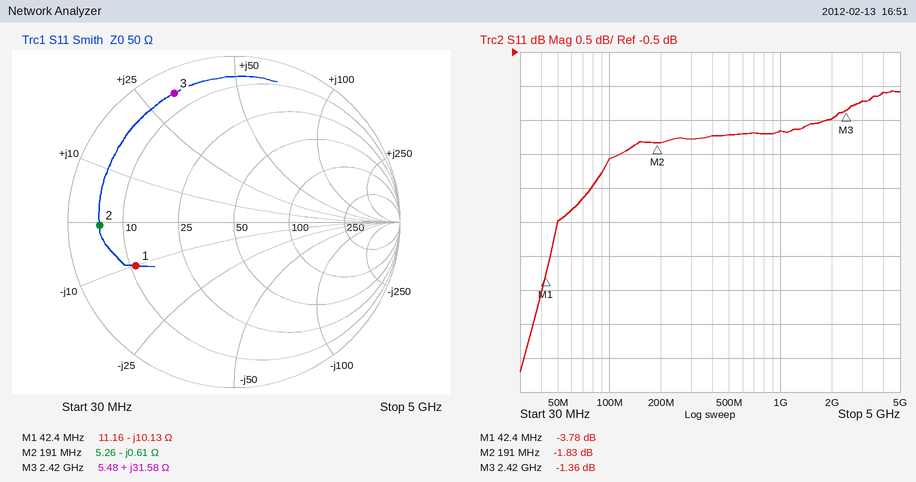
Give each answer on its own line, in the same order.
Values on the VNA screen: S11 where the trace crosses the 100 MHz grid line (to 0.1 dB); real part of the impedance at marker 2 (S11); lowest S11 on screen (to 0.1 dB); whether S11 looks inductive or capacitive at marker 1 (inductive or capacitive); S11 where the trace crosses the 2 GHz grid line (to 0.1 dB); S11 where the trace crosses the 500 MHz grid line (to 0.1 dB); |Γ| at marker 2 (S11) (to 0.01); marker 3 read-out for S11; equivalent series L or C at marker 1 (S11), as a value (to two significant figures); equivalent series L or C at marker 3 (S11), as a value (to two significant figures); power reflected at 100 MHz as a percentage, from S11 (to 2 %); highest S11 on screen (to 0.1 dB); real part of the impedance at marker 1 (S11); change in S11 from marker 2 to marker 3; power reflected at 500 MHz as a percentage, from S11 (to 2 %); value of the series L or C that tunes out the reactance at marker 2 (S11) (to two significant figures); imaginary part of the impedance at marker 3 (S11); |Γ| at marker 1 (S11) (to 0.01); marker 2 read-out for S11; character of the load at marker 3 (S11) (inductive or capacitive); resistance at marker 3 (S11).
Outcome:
-2.1 dB
5.26 Ω
-5.2 dB
capacitive
-1.5 dB
-1.7 dB
0.81
-1.36 dB
370 pF
2.1 nH
62 %
-1.1 dB
11.16 Ω
0.47 dB
68 %
510 pH
+31.58 Ω
0.65
-1.83 dB
inductive
5.48 Ω
